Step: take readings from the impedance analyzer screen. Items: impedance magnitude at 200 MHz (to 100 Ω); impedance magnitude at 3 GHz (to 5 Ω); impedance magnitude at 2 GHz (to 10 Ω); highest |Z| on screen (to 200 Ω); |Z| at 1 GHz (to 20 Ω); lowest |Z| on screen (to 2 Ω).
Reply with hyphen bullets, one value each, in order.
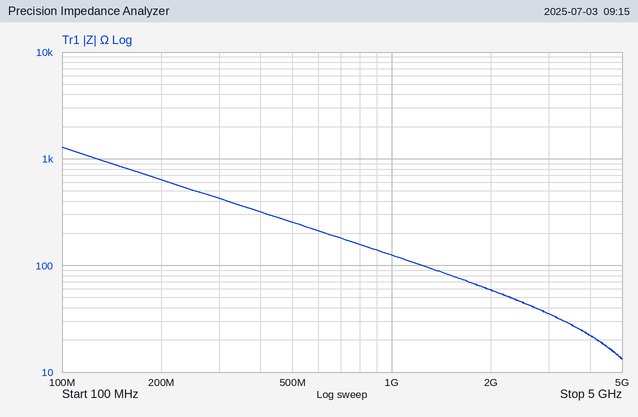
- 600 Ω
- 35 Ω
- 60 Ω
- 1.2 kΩ
- 120 Ω
- 14 Ω
